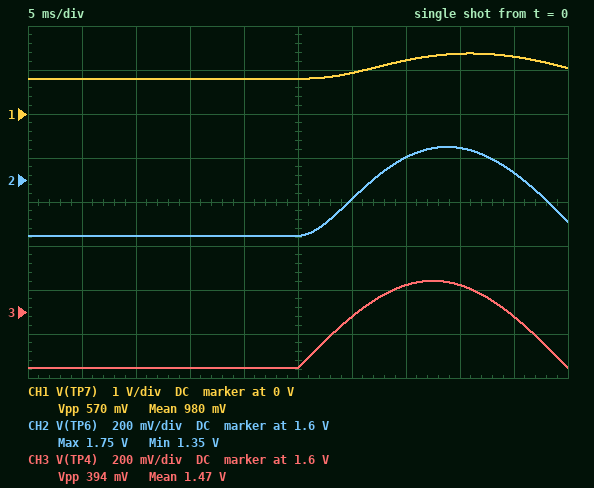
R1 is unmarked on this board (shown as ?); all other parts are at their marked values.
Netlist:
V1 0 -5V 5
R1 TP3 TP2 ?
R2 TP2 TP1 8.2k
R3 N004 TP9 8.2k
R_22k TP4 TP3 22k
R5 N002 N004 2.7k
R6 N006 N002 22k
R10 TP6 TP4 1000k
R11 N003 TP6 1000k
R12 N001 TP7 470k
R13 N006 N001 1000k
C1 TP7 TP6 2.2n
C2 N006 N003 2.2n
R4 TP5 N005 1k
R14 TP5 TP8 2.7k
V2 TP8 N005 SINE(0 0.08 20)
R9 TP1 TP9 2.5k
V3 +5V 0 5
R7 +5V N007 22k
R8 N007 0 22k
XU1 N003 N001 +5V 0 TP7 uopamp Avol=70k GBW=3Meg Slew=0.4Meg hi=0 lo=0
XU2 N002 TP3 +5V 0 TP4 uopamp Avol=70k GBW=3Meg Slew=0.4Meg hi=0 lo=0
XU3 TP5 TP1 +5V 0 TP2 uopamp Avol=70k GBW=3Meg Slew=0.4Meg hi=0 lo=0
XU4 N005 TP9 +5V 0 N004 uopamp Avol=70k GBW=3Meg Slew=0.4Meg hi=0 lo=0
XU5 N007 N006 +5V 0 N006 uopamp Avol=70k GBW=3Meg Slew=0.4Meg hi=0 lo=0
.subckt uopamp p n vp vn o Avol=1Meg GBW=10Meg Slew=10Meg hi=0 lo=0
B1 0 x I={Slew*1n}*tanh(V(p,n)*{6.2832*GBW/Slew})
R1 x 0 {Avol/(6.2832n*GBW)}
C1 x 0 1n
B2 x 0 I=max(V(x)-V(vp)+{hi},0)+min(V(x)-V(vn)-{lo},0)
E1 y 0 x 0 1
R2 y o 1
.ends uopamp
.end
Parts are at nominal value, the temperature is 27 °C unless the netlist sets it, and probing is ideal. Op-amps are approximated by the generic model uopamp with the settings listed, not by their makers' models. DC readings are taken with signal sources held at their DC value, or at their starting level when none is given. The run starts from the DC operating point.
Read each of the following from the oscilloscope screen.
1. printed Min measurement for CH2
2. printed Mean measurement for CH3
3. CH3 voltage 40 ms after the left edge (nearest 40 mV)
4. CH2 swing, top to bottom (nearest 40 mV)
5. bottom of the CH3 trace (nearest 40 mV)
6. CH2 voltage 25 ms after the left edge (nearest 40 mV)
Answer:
1.35 V
1.47 V
1.72 V
400 mV
1.36 V
1.36 V
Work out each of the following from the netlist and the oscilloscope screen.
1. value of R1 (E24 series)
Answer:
5.6 kΩ
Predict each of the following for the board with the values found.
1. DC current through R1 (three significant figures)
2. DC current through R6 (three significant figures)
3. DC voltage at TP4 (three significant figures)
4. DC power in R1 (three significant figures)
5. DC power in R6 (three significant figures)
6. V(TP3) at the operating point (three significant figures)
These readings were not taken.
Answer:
48.8 µA
101 µA
1.35 V
13.3 µW
225 µW
273 mV
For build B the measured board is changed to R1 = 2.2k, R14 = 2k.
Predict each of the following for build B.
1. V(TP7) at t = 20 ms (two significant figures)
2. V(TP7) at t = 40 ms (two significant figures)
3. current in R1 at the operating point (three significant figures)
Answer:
3.2 V
4.6 V
124 µA
